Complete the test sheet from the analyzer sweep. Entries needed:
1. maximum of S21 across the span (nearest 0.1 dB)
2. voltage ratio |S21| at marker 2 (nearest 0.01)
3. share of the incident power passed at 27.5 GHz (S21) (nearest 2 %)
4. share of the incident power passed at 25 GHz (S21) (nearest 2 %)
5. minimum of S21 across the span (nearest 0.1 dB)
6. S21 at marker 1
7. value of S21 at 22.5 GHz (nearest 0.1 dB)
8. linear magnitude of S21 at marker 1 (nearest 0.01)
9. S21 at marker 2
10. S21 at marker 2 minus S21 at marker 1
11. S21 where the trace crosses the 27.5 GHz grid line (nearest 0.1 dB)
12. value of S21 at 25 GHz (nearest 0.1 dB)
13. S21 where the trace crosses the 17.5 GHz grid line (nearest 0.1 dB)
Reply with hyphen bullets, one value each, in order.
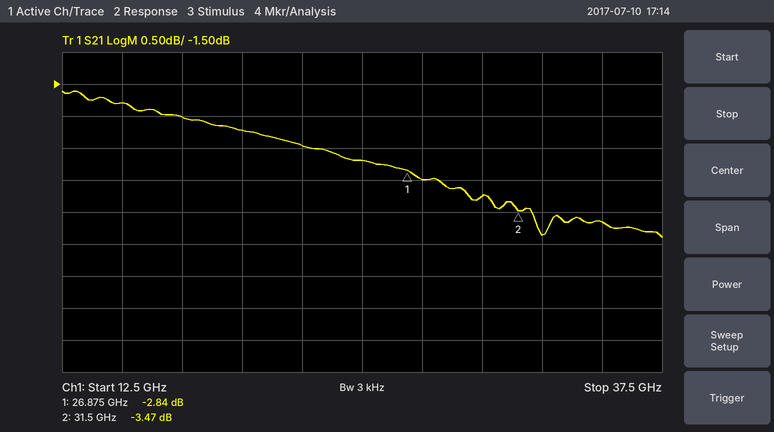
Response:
- -1.6 dB
- 0.67
- 50 %
- 54 %
- -3.9 dB
- -2.84 dB
- -2.5 dB
- 0.72
- -3.47 dB
- -0.63 dB
- -3.0 dB
- -2.7 dB
- -2.0 dB
